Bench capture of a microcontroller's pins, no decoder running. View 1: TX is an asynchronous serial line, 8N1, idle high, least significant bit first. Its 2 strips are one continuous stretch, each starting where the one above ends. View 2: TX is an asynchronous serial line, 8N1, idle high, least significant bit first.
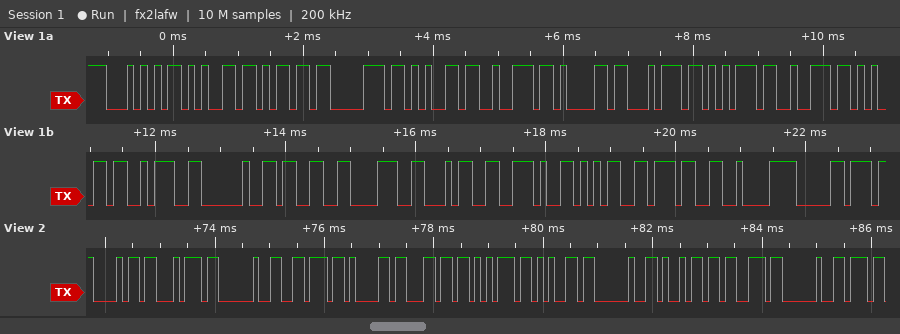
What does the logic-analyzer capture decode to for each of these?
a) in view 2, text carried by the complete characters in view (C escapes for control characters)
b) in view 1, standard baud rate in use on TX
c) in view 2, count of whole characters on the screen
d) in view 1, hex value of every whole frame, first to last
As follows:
"ht value is "
9600 baud
12
54 65 6D 70 65 72 61 74 75 72 65 3A 20 33 38 34 2E 35 37 C2 B0
